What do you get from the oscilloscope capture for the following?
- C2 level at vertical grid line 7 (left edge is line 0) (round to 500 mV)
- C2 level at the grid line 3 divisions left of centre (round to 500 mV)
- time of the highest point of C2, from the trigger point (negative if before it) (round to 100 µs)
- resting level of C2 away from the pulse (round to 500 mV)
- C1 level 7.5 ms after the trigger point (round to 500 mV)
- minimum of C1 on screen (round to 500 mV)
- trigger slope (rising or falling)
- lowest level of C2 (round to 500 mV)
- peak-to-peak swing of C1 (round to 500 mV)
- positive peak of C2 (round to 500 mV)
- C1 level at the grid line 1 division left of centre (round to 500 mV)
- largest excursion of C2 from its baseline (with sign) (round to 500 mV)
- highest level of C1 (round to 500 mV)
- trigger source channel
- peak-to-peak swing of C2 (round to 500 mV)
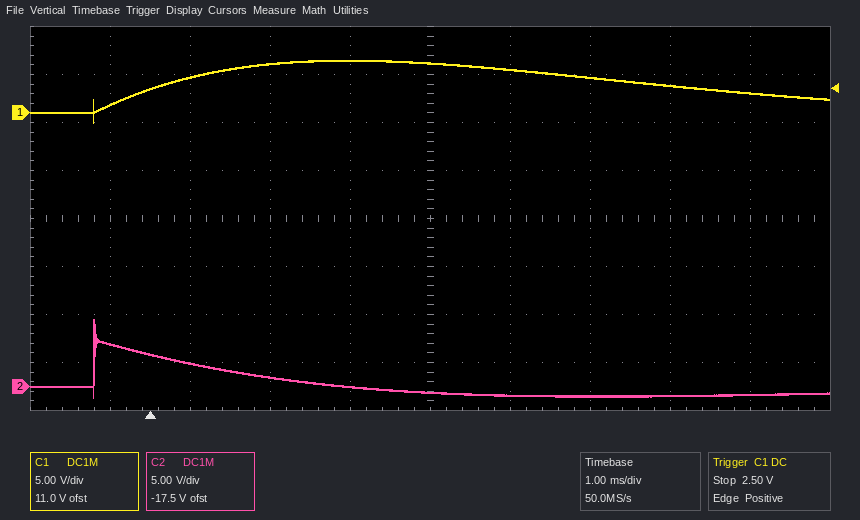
-1.0 V
2.5 V
-700 µs
-1.0 V
2.0 V
-1.0 V
rising
-1.0 V
6.5 V
7.0 V
5.5 V
+8.0 V
5.5 V
C1
8.0 V
